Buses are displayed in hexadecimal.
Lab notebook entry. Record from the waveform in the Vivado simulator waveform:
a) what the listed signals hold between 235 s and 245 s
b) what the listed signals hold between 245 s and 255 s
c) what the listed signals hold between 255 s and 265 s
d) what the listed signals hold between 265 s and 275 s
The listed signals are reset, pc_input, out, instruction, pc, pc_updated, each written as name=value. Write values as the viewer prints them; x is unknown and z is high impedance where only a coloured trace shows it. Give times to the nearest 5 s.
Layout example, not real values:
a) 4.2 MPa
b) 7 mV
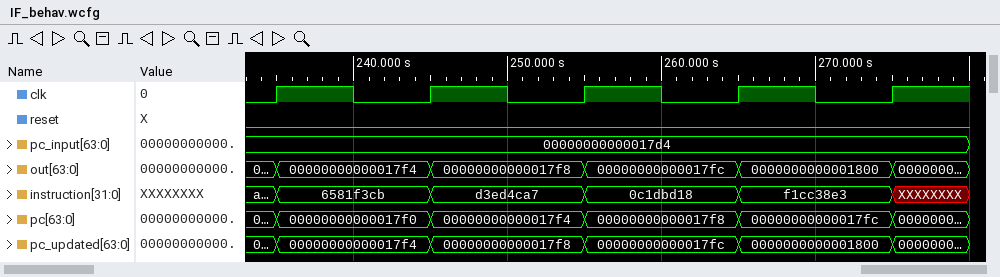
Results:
a) reset=0, pc_input=00000000000017d4, out=00000000000017f4, instruction=6581f3cb, pc=00000000000017f0, pc_updated=00000000000017f4
b) reset=0, pc_input=00000000000017d4, out=00000000000017f8, instruction=d3ed4ca7, pc=00000000000017f4, pc_updated=00000000000017f8
c) reset=0, pc_input=00000000000017d4, out=00000000000017fc, instruction=0c1dbd18, pc=00000000000017f8, pc_updated=00000000000017fc
d) reset=0, pc_input=00000000000017d4, out=0000000000001800, instruction=f1cc38e3, pc=00000000000017fc, pc_updated=0000000000001800
